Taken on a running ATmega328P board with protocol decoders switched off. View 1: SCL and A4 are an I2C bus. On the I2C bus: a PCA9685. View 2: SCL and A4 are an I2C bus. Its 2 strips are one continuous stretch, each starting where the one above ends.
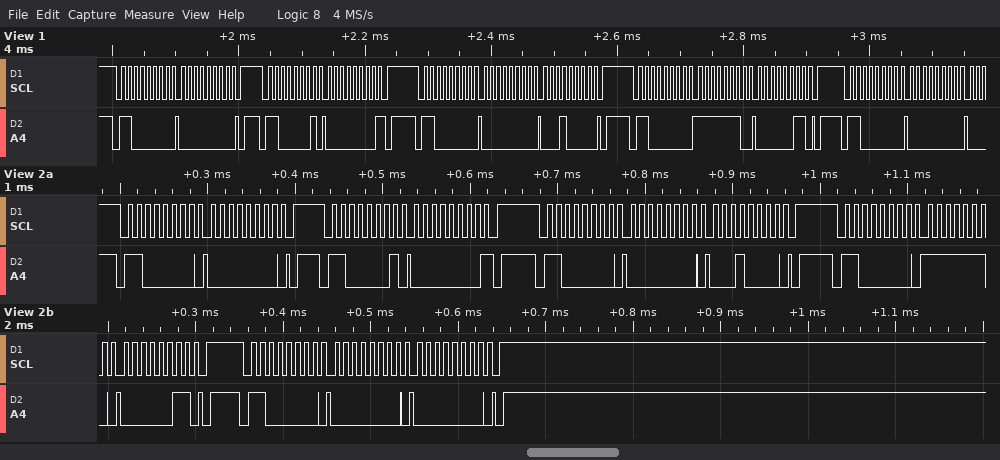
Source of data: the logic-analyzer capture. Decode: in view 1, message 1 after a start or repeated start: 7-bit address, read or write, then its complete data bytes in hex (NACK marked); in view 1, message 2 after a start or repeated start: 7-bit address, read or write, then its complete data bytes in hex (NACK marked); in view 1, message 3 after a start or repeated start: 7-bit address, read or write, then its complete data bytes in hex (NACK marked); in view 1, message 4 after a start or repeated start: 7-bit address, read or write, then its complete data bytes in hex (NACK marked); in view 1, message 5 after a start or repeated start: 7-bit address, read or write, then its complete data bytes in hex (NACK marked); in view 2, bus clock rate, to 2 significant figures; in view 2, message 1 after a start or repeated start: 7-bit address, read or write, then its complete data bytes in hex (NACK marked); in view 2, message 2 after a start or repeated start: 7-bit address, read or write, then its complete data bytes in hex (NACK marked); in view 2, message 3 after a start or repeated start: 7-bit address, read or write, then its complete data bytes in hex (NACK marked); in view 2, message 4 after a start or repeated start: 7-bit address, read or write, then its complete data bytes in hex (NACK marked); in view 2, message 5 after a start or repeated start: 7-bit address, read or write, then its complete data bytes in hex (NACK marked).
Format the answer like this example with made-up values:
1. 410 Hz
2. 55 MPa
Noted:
1. 0x60 write: 00
2. 0x60 read: 00 NACK
3. 0x60 write: 00 10
4. 0x60 write: FE 03
5. 0x60 write: 00
6. 100 kHz
7. 0x60 write: 00
8. 0x60 read: 00 NACK
9. 0x60 write: 00 10
10. 0x60 write: FE 03
11. 0x60 write: 00 00
